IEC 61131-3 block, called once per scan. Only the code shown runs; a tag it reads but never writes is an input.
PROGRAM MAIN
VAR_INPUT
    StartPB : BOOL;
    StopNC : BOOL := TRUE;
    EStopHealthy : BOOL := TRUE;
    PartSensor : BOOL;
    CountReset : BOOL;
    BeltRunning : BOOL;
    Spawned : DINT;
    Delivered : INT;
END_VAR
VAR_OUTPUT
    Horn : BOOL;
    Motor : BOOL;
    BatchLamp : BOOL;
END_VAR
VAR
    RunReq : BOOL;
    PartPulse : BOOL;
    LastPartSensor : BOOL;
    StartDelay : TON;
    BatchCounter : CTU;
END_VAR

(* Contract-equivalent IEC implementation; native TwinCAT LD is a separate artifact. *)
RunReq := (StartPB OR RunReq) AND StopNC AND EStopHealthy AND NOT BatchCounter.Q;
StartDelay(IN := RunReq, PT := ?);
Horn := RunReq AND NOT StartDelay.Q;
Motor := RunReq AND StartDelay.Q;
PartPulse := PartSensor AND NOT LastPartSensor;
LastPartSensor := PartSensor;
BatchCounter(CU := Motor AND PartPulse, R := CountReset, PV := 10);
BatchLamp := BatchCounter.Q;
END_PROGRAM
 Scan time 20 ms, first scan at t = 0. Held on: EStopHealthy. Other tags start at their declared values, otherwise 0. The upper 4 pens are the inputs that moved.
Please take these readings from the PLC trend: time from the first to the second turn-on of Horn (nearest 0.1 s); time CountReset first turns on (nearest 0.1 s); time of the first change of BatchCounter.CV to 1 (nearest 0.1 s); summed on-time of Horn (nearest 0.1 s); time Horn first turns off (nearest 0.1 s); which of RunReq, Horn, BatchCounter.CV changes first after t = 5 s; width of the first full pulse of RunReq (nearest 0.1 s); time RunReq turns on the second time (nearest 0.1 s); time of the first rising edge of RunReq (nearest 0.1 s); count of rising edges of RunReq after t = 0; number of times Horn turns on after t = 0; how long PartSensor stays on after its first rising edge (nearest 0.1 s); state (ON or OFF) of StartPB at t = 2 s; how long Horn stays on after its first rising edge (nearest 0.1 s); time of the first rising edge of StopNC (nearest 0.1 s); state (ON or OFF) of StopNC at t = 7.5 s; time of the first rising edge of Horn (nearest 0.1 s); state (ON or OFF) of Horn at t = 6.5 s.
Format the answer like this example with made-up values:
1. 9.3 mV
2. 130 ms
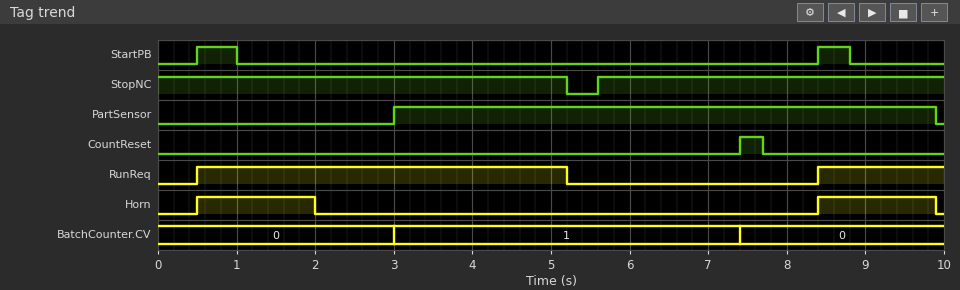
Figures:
1. 7.9 s
2. 7.4 s
3. 3.0 s
4. 3.0 s
5. 2.0 s
6. RunReq
7. 4.7 s
8. 8.4 s
9. 0.5 s
10. 2
11. 2
12. 6.9 s
13. OFF
14. 1.5 s
15. 5.6 s
16. ON
17. 0.5 s
18. OFF
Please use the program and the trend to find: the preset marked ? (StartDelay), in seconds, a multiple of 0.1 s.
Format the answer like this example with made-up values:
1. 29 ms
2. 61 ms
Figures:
1. 1.5 s
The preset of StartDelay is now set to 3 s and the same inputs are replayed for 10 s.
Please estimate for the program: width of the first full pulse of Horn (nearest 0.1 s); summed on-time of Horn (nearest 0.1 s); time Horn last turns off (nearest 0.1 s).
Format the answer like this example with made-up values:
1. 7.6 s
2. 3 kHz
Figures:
1. 3.0 s
2. 4.6 s
3. 3.5 s
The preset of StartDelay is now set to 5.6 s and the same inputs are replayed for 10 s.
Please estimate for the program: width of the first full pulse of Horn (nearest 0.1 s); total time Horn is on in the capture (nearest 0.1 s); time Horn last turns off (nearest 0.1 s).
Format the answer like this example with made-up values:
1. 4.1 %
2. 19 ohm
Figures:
1. 4.7 s
2. 6.3 s
3. 5.2 s
